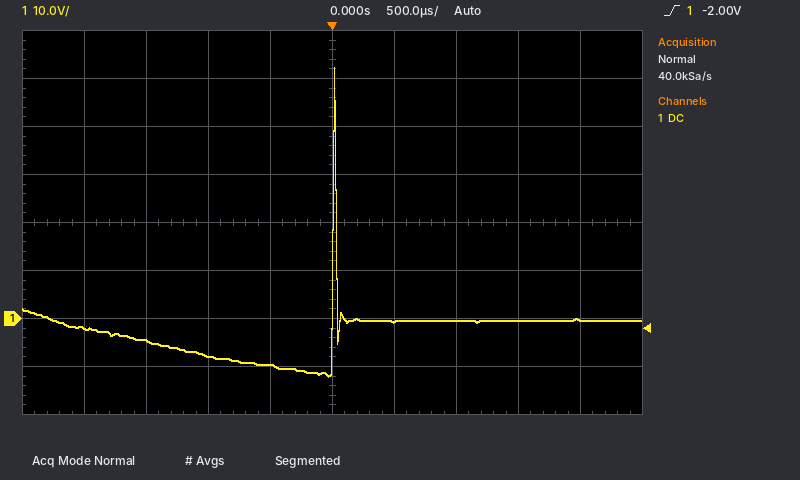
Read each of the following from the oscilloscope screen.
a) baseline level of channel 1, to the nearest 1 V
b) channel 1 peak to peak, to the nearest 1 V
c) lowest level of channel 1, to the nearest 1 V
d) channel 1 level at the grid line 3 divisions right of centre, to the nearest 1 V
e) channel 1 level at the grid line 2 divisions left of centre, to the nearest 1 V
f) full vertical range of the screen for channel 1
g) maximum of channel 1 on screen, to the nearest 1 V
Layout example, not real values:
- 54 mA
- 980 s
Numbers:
- 0 V
- 64 V
- -12 V
- 0 V
- -8 V
- 80 V
- 52 V
